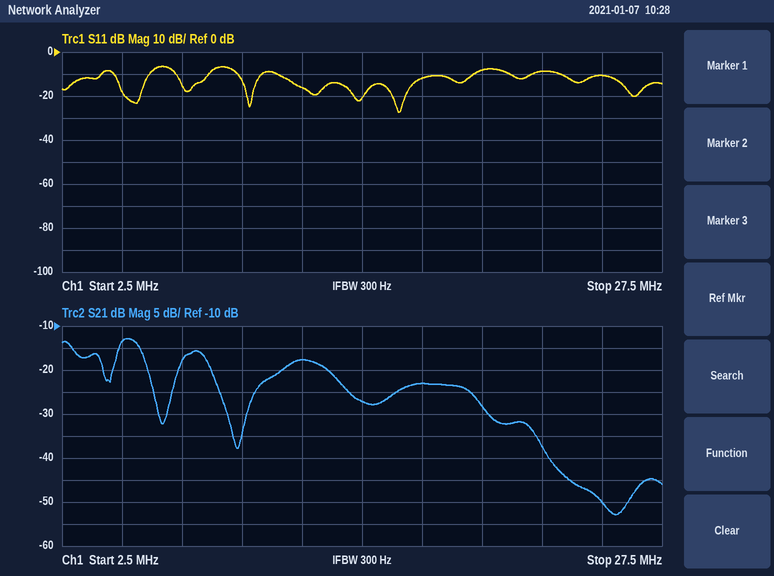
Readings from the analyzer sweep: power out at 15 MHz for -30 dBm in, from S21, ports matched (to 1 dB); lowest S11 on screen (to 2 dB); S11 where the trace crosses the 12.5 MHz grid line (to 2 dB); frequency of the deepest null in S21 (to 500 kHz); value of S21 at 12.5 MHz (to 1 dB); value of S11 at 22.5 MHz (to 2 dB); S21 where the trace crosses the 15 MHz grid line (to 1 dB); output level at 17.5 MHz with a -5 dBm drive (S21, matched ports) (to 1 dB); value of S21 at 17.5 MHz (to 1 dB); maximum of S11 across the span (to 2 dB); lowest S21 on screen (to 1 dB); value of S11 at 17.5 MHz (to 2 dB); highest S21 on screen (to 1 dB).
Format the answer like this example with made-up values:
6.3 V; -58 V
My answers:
-57 dBm; -28 dB; -16 dB; 25.5 MHz; -18 dB; -8 dB; -27 dB; -28 dBm; -23 dB; -6 dB; -53 dB; -12 dB; -13 dB
